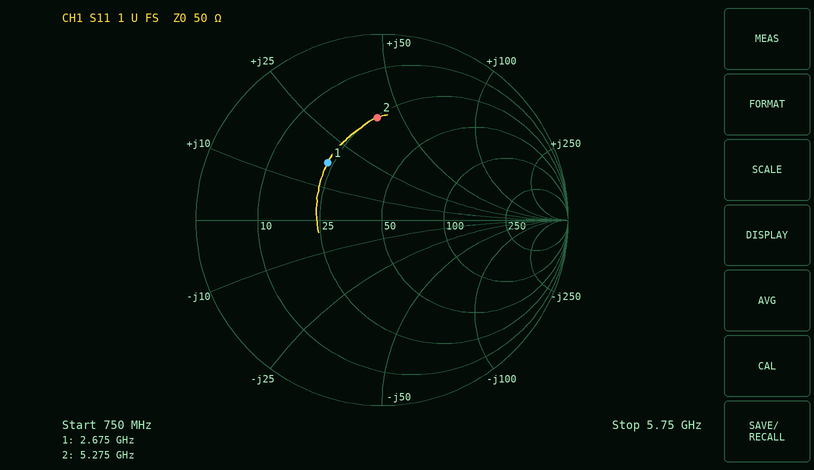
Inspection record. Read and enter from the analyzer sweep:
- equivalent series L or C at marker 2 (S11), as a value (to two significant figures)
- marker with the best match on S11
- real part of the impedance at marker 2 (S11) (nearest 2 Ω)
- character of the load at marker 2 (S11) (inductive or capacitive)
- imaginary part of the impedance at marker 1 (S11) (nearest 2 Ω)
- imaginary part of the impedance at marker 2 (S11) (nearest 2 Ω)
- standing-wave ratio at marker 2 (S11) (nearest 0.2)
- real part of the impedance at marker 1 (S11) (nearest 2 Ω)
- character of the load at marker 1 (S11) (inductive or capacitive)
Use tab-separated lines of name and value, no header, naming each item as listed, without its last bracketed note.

equivalent series L or C at marker 2 (S11), as a value	1.2 nH
marker with the best match on S11	marker 1
real part of the impedance at marker 2 (S11)	26 Ω
character of the load at marker 2 (S11)	inductive
imaginary part of the impedance at marker 1 (S11)	+18 Ω
imaginary part of the impedance at marker 2 (S11)	+40 Ω
standing-wave ratio at marker 2 (S11)	3.4
real part of the impedance at marker 1 (S11)	24 Ω
character of the load at marker 1 (S11)	inductive
